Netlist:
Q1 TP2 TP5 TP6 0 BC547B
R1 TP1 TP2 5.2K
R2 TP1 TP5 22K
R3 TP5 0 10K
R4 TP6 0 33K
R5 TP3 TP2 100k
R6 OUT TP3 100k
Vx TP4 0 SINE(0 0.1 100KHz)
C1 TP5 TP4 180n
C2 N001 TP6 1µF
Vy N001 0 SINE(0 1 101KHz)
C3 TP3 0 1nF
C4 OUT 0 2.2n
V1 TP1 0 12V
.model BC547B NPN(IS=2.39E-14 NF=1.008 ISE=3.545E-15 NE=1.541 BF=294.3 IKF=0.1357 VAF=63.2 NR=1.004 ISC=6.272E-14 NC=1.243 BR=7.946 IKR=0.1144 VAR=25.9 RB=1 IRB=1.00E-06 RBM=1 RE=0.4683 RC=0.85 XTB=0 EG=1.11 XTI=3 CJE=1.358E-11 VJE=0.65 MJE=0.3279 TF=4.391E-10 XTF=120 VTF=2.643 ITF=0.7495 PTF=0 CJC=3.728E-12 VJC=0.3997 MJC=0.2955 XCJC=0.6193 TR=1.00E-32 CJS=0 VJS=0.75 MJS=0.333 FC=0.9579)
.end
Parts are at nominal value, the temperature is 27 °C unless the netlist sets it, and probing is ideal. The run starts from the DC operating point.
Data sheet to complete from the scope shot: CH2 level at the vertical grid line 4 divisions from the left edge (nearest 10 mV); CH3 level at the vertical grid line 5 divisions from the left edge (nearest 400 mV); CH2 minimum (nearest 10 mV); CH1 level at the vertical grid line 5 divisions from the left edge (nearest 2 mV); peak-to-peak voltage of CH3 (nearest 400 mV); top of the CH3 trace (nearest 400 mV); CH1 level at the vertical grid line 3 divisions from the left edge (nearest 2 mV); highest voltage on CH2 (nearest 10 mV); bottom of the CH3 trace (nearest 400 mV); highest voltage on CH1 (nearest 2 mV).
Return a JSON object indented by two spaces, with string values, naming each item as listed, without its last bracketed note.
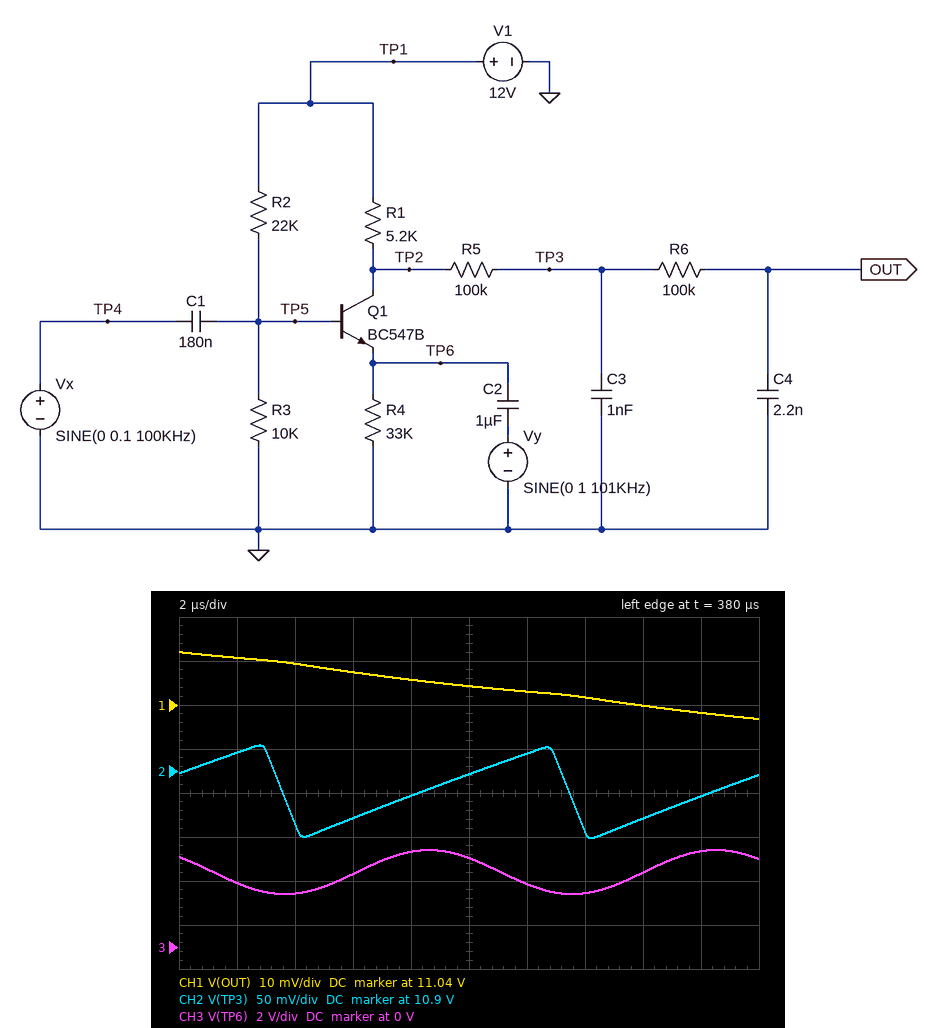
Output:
{
  "CH2 level at the vertical grid line 4 divisions from the left edge": "10.87 V",
  "CH3 level at the vertical grid line 5 divisions from the left edge": "4.0 V",
  "CH2 minimum": "10.82 V",
  "CH1 level at the vertical grid line 5 divisions from the left edge": "11.044 V",
  "peak-to-peak voltage of CH3": "2.0 V",
  "top of the CH3 trace": "4.4 V",
  "CH1 level at the vertical grid line 3 divisions from the left edge": "11.048 V",
  "highest voltage on CH2": "10.93 V",
  "bottom of the CH3 trace": "2.4 V",
  "highest voltage on CH1": "11.052 V"
}
